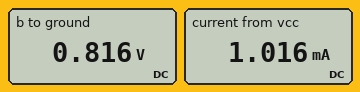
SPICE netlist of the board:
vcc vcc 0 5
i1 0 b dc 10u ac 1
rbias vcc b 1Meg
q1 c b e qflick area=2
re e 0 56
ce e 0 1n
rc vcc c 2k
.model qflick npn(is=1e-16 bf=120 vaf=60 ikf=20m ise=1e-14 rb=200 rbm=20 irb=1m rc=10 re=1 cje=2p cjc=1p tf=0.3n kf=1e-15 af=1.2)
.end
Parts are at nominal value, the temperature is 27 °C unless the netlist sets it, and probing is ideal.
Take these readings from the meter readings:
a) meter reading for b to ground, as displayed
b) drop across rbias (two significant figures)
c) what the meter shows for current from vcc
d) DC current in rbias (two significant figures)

0.816 V
4.2 V
1.016 mA
4.2 µA
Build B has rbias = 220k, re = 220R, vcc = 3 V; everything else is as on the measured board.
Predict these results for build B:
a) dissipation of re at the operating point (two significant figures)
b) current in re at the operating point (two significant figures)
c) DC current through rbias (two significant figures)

360 µW
1.3 mA
8.9 µA
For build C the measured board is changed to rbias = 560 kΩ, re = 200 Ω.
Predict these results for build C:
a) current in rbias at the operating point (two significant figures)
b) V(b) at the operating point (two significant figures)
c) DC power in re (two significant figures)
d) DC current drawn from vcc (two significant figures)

7.1 µA
1.0 V
310 µW
1.2 mA
